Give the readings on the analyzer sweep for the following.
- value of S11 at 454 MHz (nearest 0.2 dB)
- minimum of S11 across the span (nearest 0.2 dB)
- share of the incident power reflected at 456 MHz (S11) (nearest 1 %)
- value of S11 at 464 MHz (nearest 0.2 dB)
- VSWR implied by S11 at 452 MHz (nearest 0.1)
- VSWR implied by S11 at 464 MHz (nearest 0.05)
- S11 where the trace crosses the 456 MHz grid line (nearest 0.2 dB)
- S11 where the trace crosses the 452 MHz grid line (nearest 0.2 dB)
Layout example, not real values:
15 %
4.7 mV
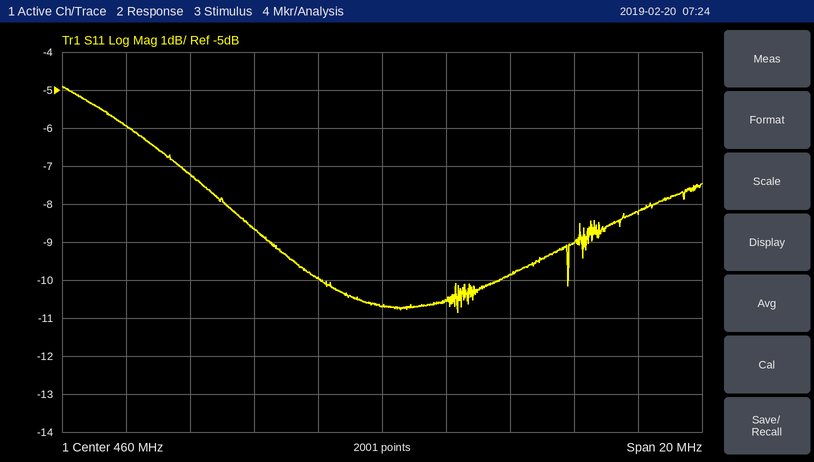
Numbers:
-7.2 dB
-10.8 dB
14 %
-9.8 dB
3.0
1.95
-8.6 dB
-6.0 dB
